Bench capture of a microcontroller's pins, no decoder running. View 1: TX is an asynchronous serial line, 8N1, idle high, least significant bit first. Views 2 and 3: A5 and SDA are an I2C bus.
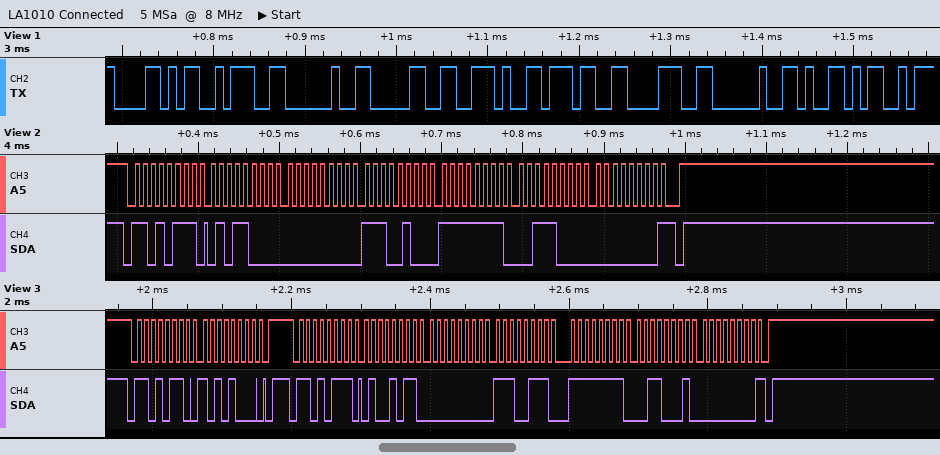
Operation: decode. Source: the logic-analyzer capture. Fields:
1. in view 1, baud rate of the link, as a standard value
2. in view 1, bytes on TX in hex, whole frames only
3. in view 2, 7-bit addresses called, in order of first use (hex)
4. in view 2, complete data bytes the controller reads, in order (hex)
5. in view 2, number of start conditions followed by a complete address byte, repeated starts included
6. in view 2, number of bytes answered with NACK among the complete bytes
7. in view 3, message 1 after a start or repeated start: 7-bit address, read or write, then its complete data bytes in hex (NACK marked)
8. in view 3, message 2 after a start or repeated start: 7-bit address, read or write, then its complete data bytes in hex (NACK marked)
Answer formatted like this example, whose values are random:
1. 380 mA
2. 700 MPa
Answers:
1. 115200 baud
2. 0x58 0x3A 0x20 0x30 0x2E 0x37 0x38 0x20 0x59
3. 0x6B
4. 58 00 E4 FF 38 00
5. 1
6. 1
7. 0x6B write: A8
8. 0x6B read: 4B 00 E7 FF 31 00 NACK
